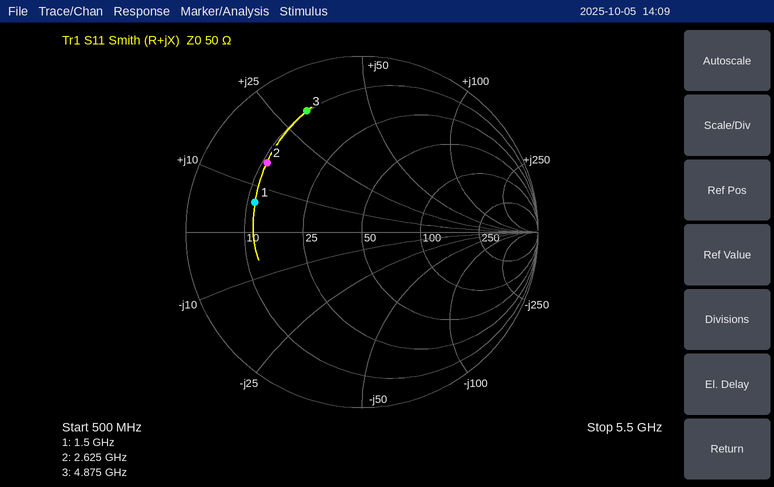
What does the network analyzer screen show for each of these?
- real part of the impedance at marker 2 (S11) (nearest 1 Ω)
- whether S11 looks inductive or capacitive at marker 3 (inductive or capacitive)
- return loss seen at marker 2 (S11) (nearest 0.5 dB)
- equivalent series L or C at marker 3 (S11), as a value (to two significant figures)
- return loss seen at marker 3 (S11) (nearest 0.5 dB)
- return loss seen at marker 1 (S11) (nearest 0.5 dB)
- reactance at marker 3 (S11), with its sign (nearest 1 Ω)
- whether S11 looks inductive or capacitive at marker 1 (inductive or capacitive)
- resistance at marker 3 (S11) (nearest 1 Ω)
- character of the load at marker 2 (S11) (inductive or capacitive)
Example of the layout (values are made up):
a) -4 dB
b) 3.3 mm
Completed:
a) 11 Ω
b) inductive
c) 3.5 dB
d) 1.0 nH
e) 2.5 dB
f) 4.0 dB
g) +31 Ω
h) inductive
i) 10 Ω
j) inductive
